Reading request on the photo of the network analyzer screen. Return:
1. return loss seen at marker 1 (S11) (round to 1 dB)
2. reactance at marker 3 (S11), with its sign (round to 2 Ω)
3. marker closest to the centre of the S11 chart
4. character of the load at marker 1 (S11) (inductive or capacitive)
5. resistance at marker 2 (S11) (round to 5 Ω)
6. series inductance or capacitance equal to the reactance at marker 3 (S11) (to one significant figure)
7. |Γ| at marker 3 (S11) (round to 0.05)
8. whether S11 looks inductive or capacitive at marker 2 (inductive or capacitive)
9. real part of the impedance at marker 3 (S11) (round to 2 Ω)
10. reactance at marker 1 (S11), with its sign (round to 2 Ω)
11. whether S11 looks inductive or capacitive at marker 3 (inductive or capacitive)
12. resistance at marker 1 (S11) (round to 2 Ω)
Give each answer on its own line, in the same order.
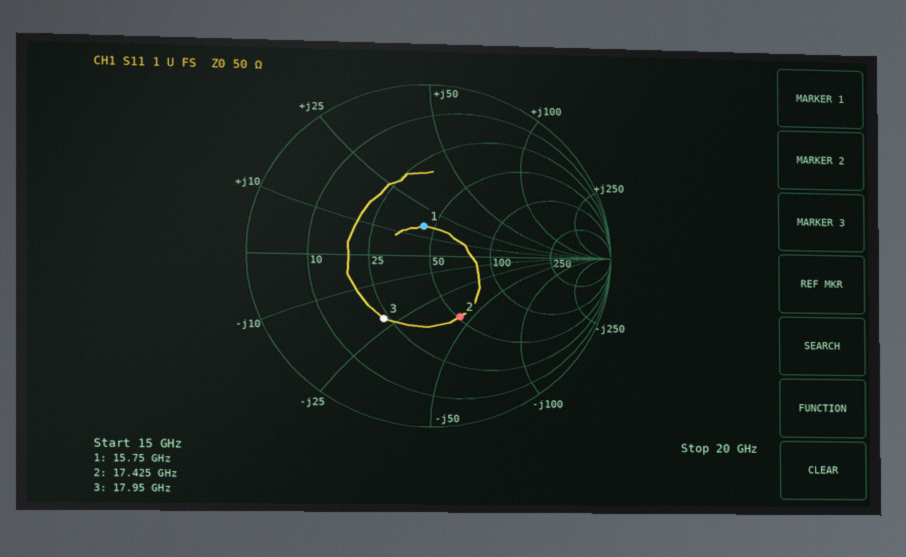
15 dB
-22 Ω
marker 1
inductive
50 Ω
400 fF
0.45
capacitive
24 Ω
+16 Ω
capacitive
44 Ω
